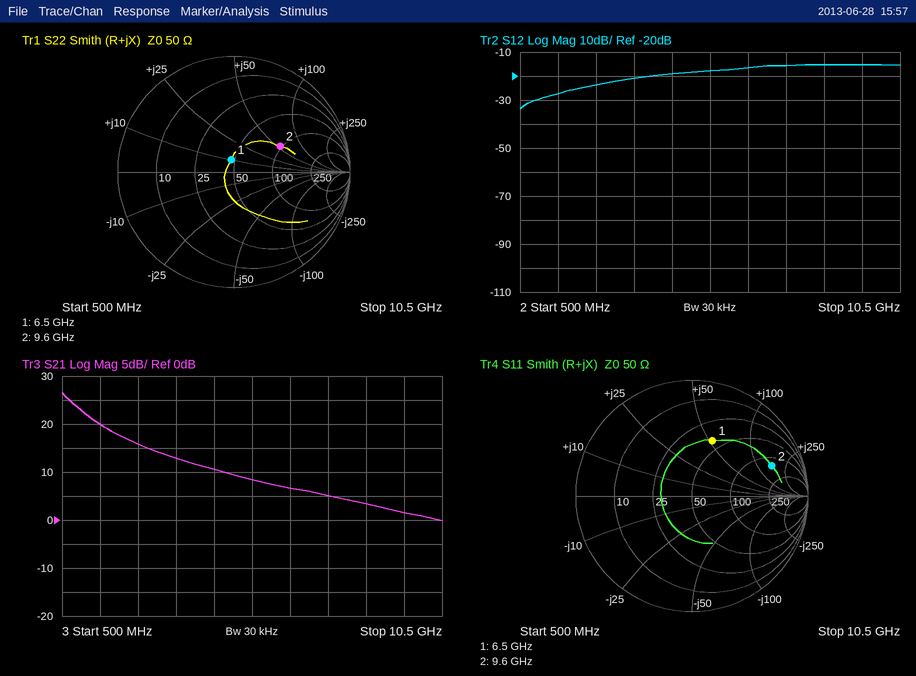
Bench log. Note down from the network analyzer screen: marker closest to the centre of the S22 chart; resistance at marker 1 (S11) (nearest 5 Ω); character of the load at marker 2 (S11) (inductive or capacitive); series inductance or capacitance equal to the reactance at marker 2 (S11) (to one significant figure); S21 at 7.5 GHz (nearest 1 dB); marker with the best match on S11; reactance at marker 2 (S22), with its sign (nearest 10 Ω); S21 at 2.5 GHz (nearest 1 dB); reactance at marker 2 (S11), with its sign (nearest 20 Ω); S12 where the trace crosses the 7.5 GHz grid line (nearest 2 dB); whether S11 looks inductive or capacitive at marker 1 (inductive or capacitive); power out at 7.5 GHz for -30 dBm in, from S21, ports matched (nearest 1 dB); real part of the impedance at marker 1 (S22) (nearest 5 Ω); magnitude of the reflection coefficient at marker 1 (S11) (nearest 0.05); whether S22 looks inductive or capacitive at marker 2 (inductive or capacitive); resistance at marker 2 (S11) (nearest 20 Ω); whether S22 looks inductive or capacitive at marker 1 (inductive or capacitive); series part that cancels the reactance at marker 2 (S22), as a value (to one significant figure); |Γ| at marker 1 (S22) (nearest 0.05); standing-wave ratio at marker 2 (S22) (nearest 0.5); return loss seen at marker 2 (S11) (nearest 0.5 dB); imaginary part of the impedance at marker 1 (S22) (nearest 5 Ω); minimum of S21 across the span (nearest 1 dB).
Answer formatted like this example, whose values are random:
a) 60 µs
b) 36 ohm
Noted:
a) marker 1
b) 40 Ω
c) inductive
d) 3 nH
e) 5 dB
f) marker 1
g) +50 Ω
h) 16 dB
i) +160 Ω
j) -16 dB
k) inductive
l) -25 dBm
m) 45 Ω
n) 0.50
o) inductive
p) 140 Ω
q) inductive
r) 300 fF
s) 0.10
t) 2.5
u) 2.5 dB
v) +10 Ω
w) 0 dB
